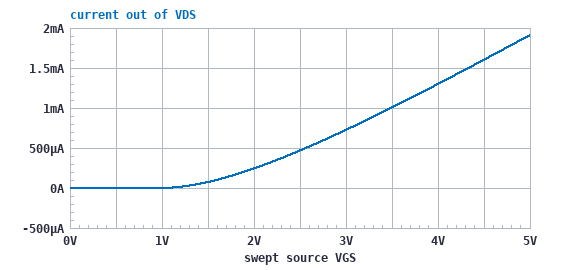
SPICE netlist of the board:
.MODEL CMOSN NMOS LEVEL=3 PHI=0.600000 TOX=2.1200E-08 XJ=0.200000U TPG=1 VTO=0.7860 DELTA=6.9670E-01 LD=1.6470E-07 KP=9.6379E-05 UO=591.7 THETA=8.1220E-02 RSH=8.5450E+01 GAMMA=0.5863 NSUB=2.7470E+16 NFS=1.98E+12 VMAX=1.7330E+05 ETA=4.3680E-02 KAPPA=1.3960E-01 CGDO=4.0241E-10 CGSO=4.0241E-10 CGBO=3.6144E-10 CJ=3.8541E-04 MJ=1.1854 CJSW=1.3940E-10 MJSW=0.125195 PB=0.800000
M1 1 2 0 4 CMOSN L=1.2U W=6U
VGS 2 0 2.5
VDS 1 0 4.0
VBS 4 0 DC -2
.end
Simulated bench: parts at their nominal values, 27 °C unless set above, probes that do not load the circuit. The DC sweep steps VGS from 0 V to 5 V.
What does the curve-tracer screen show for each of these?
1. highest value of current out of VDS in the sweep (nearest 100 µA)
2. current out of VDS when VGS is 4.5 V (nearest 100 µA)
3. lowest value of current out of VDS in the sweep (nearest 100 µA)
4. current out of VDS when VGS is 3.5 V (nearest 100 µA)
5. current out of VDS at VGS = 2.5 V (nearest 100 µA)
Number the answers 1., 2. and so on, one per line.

1. 1.9 mA
2. 1.6 mA
3. 0 A
4. 1.0 mA
5. 500 µA
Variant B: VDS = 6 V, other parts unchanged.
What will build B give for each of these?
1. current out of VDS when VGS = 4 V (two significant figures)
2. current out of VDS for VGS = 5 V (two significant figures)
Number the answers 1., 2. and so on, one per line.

1. 1.4 mA
2. 2.1 mA
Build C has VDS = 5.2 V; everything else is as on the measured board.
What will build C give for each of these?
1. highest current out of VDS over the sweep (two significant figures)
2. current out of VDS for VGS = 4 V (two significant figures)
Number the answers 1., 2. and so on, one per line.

1. 2.0 mA
2. 1.4 mA
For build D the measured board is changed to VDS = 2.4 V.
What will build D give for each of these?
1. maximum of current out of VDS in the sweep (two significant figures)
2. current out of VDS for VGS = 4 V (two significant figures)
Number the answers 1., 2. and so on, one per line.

1. 1.7 mA
2. 1.2 mA
